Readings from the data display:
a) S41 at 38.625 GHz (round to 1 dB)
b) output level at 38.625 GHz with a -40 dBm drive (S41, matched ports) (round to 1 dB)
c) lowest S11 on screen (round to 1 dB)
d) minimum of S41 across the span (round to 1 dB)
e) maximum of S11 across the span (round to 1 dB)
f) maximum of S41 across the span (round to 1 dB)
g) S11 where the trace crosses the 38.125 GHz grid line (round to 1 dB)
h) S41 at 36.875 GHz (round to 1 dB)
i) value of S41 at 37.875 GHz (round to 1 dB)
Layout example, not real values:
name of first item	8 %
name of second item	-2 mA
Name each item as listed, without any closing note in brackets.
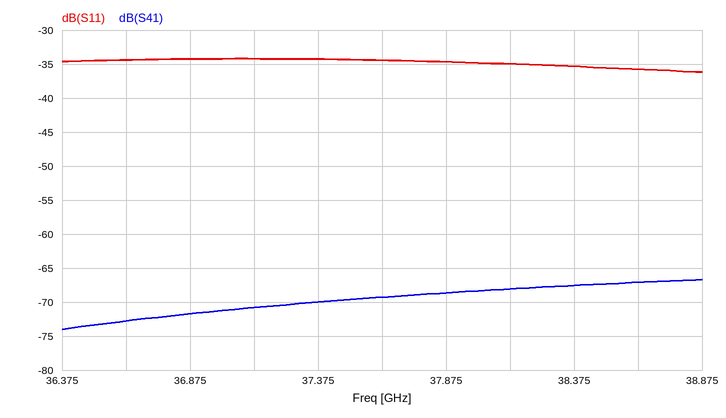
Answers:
S41 at 38.625 GHz	-67 dB
output level at 38.625 GHz with a -40 dBm drive (S41, matched ports)	-107 dBm
lowest S11 on screen	-36 dB
minimum of S41 across the span	-74 dB
maximum of S11 across the span	-34 dB
maximum of S41 across the span	-67 dB
S11 where the trace crosses the 38.125 GHz grid line	-35 dB
S41 at 36.875 GHz	-72 dB
value of S41 at 37.875 GHz	-69 dB
